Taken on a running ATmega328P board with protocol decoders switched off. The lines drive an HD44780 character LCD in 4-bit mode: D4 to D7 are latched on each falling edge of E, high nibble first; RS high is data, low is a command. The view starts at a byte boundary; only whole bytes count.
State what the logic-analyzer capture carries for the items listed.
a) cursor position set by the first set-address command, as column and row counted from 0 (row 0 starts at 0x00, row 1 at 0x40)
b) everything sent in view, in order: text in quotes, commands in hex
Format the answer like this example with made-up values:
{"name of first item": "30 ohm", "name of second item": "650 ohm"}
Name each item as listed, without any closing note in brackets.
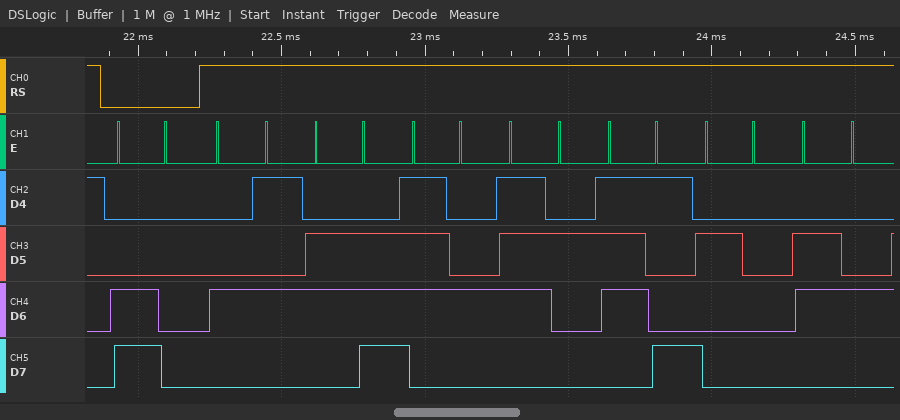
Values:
{"cursor position set by the first set-address command, as column and row counted from 0": "column 0, row 1", "everything sent in view, in order: text in quotes, commands in hex": "0xC0 \"Entry d\""}
